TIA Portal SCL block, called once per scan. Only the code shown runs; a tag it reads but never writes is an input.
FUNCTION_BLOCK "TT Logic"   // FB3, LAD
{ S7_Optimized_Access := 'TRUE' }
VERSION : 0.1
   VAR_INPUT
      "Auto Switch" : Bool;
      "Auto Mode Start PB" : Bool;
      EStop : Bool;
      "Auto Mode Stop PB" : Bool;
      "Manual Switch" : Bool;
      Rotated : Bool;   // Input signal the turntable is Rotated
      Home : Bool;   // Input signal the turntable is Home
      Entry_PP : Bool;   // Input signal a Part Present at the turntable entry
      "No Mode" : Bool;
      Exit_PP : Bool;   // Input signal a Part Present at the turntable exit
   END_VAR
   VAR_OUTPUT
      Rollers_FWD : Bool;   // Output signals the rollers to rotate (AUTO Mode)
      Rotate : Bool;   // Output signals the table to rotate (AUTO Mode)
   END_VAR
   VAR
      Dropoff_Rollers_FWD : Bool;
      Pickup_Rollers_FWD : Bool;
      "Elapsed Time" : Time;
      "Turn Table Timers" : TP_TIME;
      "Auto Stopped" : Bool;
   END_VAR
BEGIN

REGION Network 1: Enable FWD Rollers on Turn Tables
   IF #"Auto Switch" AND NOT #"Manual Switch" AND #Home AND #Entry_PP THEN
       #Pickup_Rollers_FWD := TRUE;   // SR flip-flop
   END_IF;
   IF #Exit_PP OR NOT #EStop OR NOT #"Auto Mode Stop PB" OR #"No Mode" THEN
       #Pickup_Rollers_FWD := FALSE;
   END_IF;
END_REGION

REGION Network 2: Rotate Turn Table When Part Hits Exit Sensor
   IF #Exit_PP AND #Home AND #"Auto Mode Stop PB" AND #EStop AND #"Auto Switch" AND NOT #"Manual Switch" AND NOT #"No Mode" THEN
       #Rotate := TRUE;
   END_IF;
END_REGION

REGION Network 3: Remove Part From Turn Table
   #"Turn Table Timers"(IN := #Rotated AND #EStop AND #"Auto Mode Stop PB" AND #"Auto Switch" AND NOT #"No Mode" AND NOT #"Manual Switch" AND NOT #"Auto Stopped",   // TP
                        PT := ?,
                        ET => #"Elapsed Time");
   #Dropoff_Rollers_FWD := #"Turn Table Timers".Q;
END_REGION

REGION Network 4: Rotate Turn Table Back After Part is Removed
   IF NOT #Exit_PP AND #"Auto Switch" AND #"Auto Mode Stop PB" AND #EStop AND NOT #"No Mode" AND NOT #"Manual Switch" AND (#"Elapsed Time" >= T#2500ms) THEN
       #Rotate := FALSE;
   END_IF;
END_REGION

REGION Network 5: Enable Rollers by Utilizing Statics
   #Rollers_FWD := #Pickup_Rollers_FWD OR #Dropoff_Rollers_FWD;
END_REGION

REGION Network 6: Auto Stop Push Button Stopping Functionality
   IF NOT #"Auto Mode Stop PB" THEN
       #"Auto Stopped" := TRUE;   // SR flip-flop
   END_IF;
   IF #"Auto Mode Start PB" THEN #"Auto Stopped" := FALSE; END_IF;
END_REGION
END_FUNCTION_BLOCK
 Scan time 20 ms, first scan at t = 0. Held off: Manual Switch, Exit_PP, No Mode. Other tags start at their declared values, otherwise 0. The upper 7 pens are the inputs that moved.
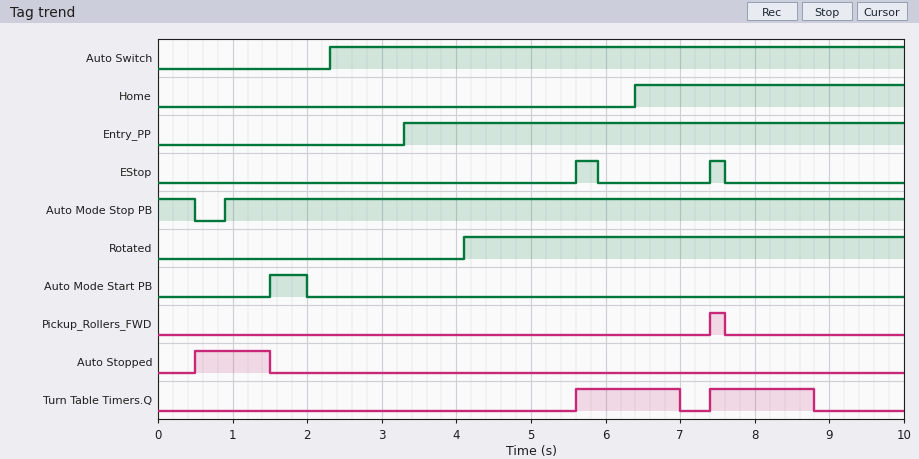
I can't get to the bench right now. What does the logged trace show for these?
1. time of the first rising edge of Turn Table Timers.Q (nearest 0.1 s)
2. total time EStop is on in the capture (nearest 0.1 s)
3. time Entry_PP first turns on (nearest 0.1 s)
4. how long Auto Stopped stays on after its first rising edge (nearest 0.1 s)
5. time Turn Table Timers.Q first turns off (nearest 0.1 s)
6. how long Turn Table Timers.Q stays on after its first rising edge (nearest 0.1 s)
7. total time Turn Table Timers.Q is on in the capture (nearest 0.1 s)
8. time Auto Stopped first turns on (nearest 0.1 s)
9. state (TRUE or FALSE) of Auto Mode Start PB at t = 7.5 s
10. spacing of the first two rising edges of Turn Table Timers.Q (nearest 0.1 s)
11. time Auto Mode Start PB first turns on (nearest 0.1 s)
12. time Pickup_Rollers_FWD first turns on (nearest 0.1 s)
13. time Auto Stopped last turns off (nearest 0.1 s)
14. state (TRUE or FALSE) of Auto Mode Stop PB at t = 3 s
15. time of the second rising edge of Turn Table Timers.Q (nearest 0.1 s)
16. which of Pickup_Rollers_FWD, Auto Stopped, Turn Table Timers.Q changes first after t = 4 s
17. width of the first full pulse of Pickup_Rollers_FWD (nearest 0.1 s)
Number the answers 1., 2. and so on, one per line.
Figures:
1. 5.6 s
2. 0.5 s
3. 3.3 s
4. 1.0 s
5. 7.0 s
6. 1.4 s
7. 2.8 s
8. 0.5 s
9. FALSE
10. 1.8 s
11. 1.5 s
12. 7.4 s
13. 1.5 s
14. TRUE
15. 7.4 s
16. Turn Table Timers.Q
17. 0.2 s
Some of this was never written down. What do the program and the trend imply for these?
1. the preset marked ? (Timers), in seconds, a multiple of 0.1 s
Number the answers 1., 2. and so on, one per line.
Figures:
1. 1.4 s
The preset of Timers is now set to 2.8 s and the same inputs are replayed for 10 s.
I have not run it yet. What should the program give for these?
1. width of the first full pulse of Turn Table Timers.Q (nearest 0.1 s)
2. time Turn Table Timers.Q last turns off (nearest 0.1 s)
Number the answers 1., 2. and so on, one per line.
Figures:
1. 2.8 s
2. 8.4 s
